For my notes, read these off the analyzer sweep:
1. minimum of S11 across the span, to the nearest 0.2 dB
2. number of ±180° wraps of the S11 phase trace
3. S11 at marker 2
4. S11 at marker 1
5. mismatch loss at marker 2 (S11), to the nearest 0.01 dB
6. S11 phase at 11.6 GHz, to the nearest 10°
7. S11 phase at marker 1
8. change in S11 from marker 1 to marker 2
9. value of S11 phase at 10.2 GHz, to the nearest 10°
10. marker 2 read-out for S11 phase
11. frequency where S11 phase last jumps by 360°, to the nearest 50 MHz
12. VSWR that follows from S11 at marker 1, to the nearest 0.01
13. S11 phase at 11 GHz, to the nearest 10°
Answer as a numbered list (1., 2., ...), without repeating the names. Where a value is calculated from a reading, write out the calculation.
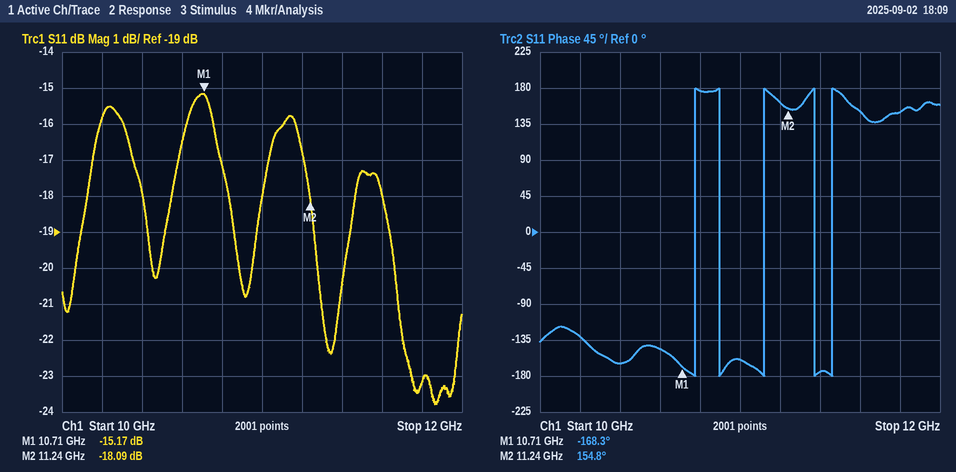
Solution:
1. -23.8 dB
2. 5
3. -18.09 dB
4. -15.17 dB
5. −10 log10(1 − 10^(-18.09/10)) ≈ 0.07 dB
6. 150°
7. -168.3°
8. -18.09 − (-15.17) = -2.92 dB
9. -130°
10. 154.8°
11. 11.45 GHz
12. (1 + 0.1744)/(1 − 0.1744) ≈ 1.42
13. -160°
